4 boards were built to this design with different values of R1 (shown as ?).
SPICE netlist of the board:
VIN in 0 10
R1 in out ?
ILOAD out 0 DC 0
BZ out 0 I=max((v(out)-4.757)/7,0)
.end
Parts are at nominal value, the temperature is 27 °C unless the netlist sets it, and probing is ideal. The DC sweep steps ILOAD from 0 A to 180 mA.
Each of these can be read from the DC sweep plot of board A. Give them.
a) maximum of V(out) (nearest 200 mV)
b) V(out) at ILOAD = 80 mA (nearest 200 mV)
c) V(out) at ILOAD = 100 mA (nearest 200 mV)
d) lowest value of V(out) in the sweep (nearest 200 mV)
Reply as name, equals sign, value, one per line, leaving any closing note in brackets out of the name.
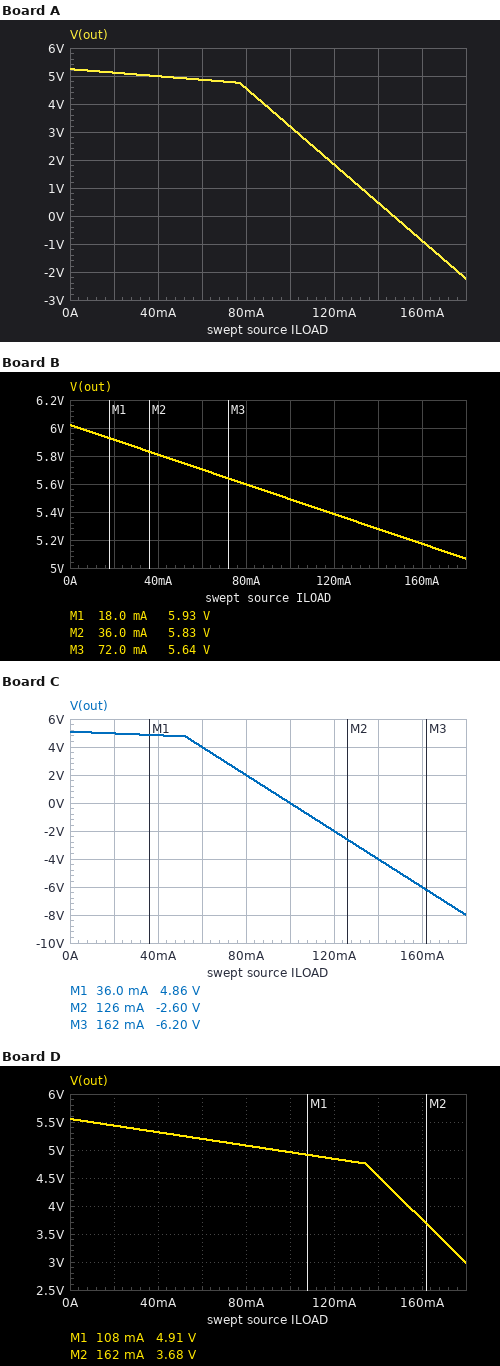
maximum of V(out) = 5.2 V
V(out) at ILOAD = 80 mA = 4.6 V
V(out) at ILOAD = 100 mA = 3.2 V
lowest value of V(out) in the sweep = -2.2 V
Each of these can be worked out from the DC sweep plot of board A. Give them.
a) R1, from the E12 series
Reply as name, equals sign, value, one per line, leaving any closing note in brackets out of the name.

R1, from the E12 series = 68 Ω
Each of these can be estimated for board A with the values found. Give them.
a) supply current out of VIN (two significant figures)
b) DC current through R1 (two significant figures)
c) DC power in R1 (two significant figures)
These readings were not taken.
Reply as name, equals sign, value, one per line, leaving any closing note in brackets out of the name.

supply current out of VIN = 70 mA
DC current through R1 = 70 mA
DC power in R1 = 330 mW
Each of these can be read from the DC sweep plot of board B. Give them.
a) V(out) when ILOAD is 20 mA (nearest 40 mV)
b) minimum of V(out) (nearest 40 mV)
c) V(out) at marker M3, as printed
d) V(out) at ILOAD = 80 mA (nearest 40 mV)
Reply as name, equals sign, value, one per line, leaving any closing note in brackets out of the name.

V(out) when ILOAD is 20 mA = 5.92 V
minimum of V(out) = 5.08 V
V(out) at marker M3, as printed = 5.64 V
V(out) at ILOAD = 80 mA = 5.60 V
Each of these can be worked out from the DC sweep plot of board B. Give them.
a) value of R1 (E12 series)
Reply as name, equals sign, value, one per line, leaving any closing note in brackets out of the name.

value of R1 = 22 Ω
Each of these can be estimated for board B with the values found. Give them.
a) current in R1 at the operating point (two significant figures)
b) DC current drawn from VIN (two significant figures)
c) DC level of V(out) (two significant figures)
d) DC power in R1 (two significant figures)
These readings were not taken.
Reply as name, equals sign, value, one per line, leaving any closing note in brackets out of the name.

current in R1 at the operating point = 180 mA
DC current drawn from VIN = 180 mA
DC level of V(out) = 6.0 V
DC power in R1 = 720 mW
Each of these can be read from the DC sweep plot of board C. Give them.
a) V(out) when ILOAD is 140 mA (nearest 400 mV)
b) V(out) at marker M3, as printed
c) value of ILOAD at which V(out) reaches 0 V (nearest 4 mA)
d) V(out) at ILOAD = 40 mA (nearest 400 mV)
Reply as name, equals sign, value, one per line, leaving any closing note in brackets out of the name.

V(out) when ILOAD is 140 mA = -4.0 V
V(out) at marker M3, as printed = -6.20 V
value of ILOAD at which V(out) reaches 0 V = 100 mA
V(out) at ILOAD = 40 mA = 4.8 V
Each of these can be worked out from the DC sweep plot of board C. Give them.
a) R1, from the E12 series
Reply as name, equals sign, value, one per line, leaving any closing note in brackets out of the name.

R1, from the E12 series = 100 Ω
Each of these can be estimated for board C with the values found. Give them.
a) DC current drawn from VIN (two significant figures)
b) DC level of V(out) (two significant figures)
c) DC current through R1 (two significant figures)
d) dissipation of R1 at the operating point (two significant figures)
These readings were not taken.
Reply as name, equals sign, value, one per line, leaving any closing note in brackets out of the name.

DC current drawn from VIN = 49 mA
DC level of V(out) = 5.1 V
DC current through R1 = 49 mA
dissipation of R1 at the operating point = 240 mW
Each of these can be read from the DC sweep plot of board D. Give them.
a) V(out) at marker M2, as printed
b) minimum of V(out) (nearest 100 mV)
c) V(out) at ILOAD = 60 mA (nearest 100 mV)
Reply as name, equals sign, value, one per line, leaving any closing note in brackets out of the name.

V(out) at marker M2, as printed = 3.68 V
minimum of V(out) = 3.0 V
V(out) at ILOAD = 60 mA = 5.2 V
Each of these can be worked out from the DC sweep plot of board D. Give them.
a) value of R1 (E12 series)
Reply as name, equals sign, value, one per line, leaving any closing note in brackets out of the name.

value of R1 = 39 Ω
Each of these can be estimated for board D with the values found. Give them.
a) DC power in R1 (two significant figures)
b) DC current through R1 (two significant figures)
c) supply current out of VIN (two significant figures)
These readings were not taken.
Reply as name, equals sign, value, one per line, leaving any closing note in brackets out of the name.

DC power in R1 = 510 mW
DC current through R1 = 110 mA
supply current out of VIN = 110 mA
